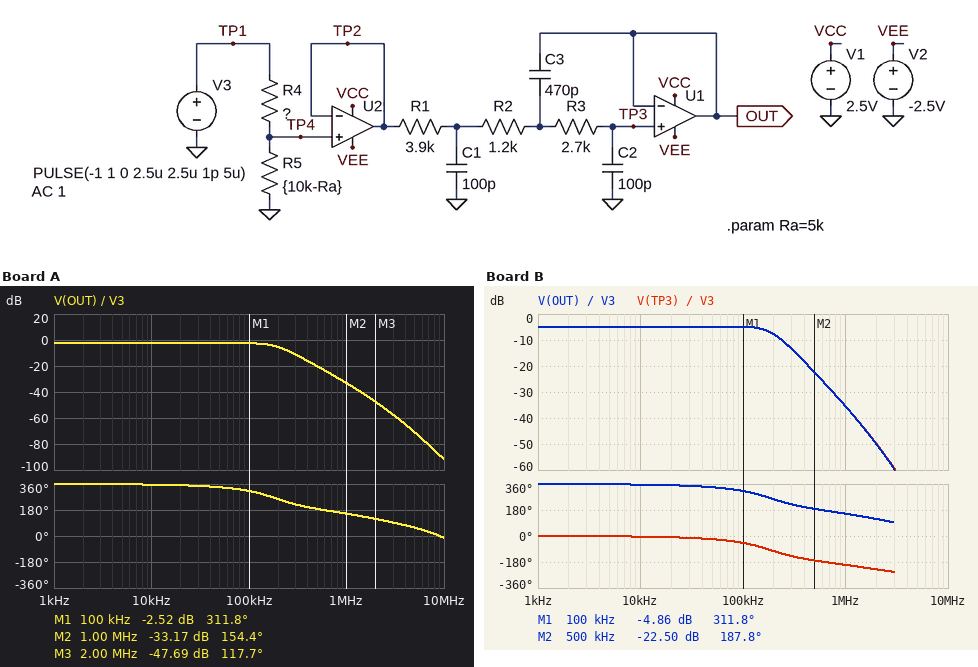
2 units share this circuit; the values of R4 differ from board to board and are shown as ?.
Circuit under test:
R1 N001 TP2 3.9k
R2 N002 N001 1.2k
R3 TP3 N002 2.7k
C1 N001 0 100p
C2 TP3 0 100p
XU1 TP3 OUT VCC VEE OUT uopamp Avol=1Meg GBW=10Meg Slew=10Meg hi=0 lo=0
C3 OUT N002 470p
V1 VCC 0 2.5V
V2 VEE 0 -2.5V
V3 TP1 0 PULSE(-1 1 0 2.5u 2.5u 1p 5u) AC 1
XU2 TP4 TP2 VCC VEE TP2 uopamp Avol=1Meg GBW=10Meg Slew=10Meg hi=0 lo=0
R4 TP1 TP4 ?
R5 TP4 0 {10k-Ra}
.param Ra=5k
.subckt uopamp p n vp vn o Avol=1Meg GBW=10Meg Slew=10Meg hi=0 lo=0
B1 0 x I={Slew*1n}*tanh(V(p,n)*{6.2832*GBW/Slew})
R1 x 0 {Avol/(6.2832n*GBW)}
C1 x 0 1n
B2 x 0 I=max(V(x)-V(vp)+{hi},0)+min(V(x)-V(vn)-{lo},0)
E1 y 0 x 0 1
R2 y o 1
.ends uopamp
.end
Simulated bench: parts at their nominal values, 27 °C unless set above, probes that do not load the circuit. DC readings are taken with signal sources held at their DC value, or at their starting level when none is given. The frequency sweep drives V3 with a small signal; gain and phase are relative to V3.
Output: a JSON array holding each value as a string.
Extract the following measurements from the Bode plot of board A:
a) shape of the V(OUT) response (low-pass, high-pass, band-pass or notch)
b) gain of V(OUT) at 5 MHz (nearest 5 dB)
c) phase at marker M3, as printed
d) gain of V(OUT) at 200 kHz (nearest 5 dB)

["low-pass", "-70 dB", "117.7 deg", "-5 dB"]
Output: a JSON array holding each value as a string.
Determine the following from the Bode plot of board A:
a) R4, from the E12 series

["1.8 kΩ"]
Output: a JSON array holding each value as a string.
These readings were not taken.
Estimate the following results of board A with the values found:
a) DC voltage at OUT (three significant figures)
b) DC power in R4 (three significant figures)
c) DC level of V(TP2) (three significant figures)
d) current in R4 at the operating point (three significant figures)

["-735 mV", "38.9 µW", "-735 mV", "147 µA"]
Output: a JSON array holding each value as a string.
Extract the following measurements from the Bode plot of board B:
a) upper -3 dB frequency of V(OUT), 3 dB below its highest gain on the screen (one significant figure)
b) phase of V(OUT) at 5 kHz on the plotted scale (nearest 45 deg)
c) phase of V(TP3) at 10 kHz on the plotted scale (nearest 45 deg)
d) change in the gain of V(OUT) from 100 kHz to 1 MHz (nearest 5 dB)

["200 kHz", "360 deg", "0 deg", "-30 dB"]
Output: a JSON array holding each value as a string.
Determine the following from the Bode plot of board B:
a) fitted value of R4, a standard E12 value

["3.9 kΩ"]
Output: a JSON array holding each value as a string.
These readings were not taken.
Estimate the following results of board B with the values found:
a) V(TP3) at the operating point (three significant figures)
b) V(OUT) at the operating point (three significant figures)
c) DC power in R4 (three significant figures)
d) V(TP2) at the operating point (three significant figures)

["-562 mV", "-562 mV", "49.2 µW", "-562 mV"]
